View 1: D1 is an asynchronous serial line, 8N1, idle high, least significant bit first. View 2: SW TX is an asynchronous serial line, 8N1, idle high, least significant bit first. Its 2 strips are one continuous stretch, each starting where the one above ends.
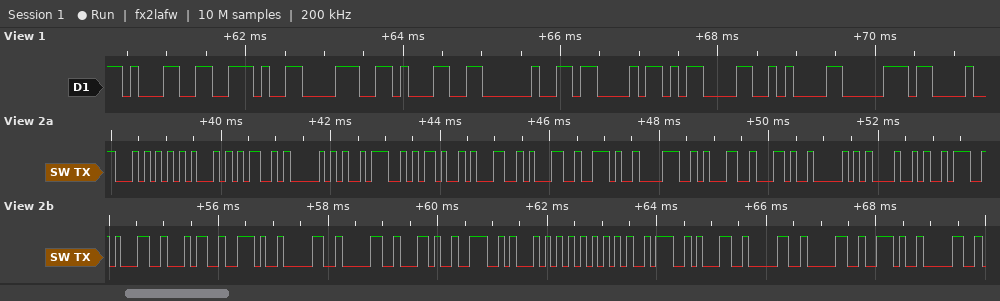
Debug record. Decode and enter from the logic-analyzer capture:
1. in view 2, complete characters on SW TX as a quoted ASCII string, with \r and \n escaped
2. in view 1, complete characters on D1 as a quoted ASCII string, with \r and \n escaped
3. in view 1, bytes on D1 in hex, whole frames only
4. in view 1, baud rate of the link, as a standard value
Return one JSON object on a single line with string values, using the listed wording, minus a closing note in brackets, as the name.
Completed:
{"in view 2, complete characters on SW TX as a quoted ASCII string, with \\r and \\n escaped": "\"TEMP:-11.81,PH:14.00,NTU:100.0\"", "in view 1, complete characters on D1 as a quoted ASCII string, with \\r and \\n escaped": "\"1.81 C\\r\\np\"", "in view 1, bytes on D1 in hex, whole frames only": "31 2E 38 31 20 43 0D 0A 70", "in view 1, baud rate of the link, as a standard value": "9600 baud"}
